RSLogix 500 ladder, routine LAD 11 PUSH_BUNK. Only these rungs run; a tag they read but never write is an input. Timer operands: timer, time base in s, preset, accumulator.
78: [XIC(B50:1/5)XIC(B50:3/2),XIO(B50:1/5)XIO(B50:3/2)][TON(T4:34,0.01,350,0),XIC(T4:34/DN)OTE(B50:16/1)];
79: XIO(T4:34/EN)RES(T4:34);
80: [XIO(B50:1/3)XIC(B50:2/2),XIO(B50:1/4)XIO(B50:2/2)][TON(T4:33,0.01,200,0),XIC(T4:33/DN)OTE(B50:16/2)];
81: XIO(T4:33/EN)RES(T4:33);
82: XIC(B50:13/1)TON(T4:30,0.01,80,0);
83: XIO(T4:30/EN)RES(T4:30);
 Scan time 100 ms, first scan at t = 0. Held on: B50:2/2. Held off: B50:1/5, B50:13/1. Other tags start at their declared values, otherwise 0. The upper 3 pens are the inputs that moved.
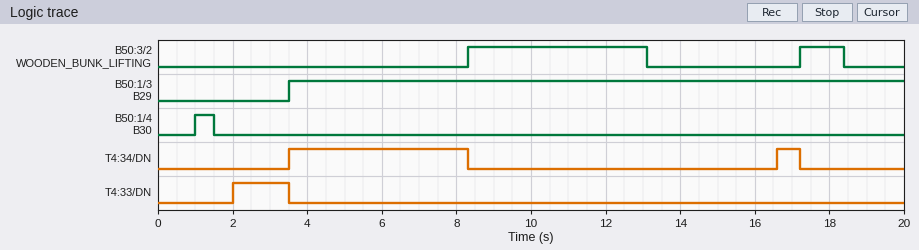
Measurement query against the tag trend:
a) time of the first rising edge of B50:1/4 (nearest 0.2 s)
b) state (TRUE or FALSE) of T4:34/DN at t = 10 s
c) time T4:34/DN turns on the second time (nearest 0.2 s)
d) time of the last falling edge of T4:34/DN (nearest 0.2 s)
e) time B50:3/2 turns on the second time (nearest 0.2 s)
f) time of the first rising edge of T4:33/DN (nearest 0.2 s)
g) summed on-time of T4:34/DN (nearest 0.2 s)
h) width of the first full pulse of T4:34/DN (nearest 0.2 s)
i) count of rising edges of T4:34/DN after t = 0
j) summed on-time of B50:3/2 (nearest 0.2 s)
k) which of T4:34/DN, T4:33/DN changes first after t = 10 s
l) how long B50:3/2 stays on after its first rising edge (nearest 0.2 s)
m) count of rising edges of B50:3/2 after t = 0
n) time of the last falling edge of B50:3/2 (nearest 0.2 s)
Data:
1.0 s
FALSE
16.6 s
17.2 s
17.2 s
2.0 s
5.4 s
4.8 s
2
6.0 s
T4:34/DN
4.8 s
2
18.4 s
